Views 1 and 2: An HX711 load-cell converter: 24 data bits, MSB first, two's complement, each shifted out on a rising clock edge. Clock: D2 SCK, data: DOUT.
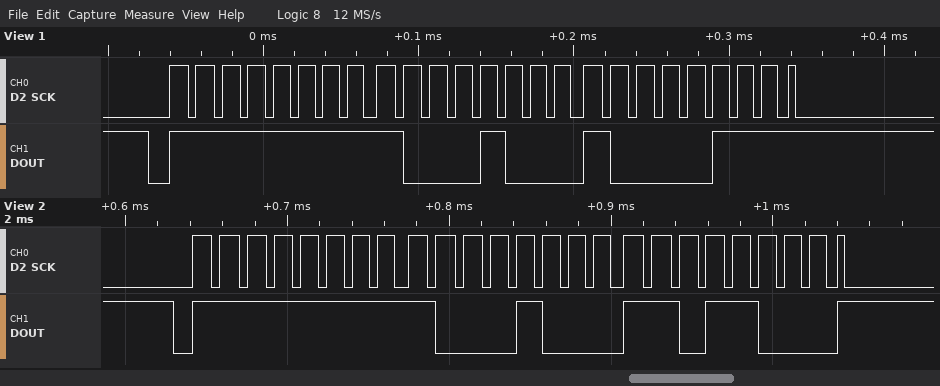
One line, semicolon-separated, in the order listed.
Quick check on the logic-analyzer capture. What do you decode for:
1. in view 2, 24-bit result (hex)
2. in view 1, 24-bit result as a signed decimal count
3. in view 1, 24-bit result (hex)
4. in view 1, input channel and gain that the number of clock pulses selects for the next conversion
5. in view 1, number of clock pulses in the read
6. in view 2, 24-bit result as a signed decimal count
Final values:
0xFF88D8; -30585; 0xFF8887; channel A, gain 128; 25; -30504
